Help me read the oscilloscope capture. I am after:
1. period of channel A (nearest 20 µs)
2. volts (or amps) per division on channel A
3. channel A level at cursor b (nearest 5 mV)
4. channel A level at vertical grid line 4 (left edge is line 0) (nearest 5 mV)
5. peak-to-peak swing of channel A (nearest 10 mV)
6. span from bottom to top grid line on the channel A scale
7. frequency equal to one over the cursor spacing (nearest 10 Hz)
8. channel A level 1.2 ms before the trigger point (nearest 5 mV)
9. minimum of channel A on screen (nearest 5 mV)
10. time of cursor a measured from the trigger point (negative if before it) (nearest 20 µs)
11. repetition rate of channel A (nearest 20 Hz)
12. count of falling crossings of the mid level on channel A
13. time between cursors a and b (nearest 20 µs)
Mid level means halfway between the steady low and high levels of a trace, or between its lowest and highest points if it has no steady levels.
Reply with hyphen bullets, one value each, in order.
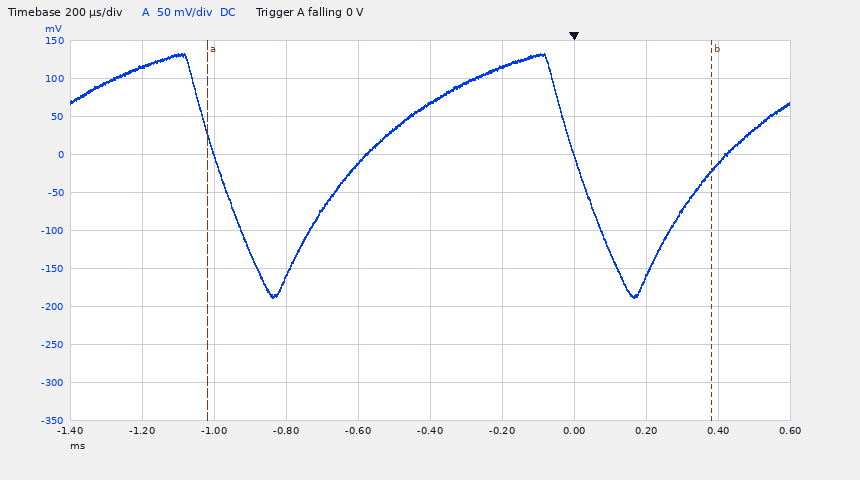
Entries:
- 1.00 ms
- 50 mV
- -20 mV
- -10 mV
- 320 mV
- 500 mV
- 710 Hz
- 115 mV
- -190 mV
- -1.02 ms
- 1.00 kHz
- 2
- 1.40 ms
